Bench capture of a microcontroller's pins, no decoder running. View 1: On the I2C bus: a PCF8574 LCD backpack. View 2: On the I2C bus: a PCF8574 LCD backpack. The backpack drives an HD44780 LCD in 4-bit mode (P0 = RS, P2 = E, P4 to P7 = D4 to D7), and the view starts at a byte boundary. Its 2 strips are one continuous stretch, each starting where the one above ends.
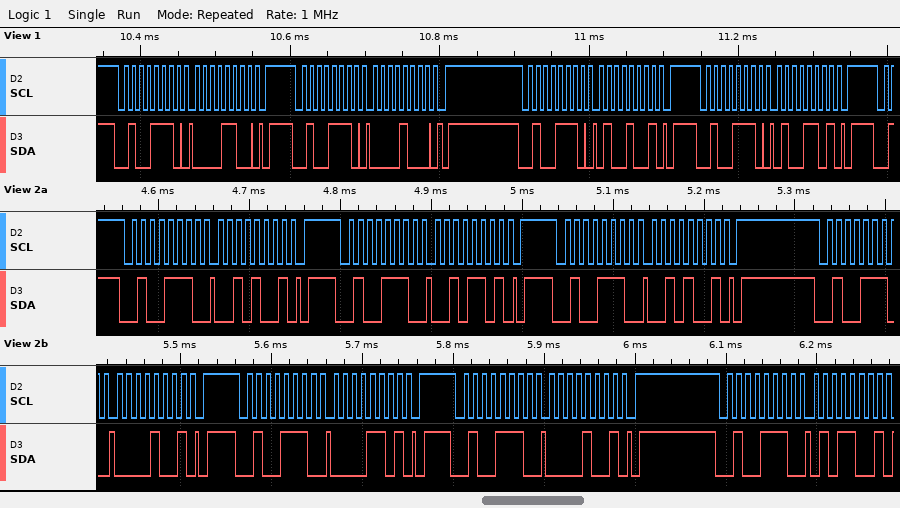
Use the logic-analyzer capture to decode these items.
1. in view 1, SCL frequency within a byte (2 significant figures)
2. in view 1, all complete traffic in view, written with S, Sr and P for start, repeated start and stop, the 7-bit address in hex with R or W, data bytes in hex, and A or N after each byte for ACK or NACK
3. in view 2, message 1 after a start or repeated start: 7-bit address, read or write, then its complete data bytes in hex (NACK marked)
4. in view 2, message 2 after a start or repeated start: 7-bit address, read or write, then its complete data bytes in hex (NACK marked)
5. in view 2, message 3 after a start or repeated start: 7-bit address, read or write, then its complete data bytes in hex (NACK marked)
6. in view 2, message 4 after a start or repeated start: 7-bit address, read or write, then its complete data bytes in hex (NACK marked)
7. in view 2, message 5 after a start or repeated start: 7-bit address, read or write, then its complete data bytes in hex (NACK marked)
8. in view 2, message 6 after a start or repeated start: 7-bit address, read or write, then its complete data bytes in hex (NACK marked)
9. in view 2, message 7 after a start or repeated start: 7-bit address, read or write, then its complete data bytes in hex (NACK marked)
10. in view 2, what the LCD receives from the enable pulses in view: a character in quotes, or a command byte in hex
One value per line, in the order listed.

100 kHz
S 27W A 0C A P S 27W A 08 A P S 27W A 49 A P S 27W A 4D A P
0x27 write: 29
0x27 write: 2D
0x27 write: 29
0x27 write: 09
0x27 write: 0D
0x27 write: 09
0x27 write: 59
' '
